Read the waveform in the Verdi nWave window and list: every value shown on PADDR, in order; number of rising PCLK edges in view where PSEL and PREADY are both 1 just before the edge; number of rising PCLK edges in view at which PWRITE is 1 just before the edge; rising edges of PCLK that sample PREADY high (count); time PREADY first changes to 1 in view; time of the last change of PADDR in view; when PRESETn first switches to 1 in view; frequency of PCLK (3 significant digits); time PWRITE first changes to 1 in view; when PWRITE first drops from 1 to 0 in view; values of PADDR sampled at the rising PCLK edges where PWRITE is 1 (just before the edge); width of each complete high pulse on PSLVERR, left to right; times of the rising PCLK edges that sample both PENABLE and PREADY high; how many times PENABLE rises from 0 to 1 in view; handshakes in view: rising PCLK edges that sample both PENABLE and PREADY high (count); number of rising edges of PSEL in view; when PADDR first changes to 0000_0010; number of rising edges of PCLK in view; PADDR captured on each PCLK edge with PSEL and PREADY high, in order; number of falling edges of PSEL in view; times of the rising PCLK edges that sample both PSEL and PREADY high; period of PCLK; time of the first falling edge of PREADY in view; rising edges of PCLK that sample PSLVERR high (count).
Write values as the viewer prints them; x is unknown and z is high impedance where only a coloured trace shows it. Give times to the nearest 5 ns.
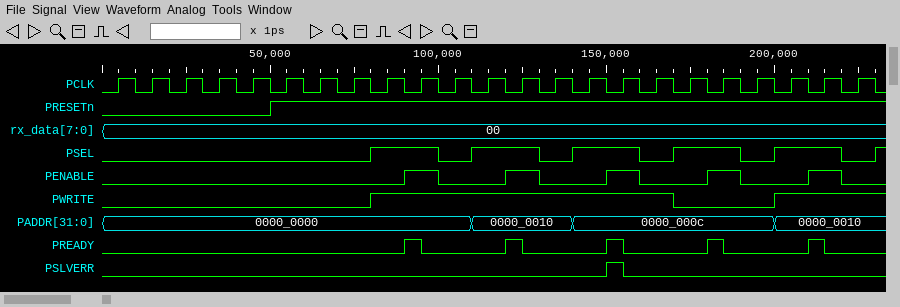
0000_0000, 0000_0010, 0000_000c, 0000_0010
5
12
5
90 ns
200 ns
50 ns
100 MHz
80 ns
170 ns
0000_0000, 0000_0000, 0000_0000, 0000_0010, 0000_0010, 0000_0010, 0000_000c, 0000_000c, 0000_000c, 0000_0010, 0000_0010, 0000_0010
5 ns
95 ns, 125 ns, 155 ns, 185 ns, 215 ns
5
5
6
110 ns
23
0000_0000, 0000_0010, 0000_000c, 0000_000c, 0000_0010
5
95 ns, 125 ns, 155 ns, 185 ns, 215 ns
10 ns
95 ns
1
